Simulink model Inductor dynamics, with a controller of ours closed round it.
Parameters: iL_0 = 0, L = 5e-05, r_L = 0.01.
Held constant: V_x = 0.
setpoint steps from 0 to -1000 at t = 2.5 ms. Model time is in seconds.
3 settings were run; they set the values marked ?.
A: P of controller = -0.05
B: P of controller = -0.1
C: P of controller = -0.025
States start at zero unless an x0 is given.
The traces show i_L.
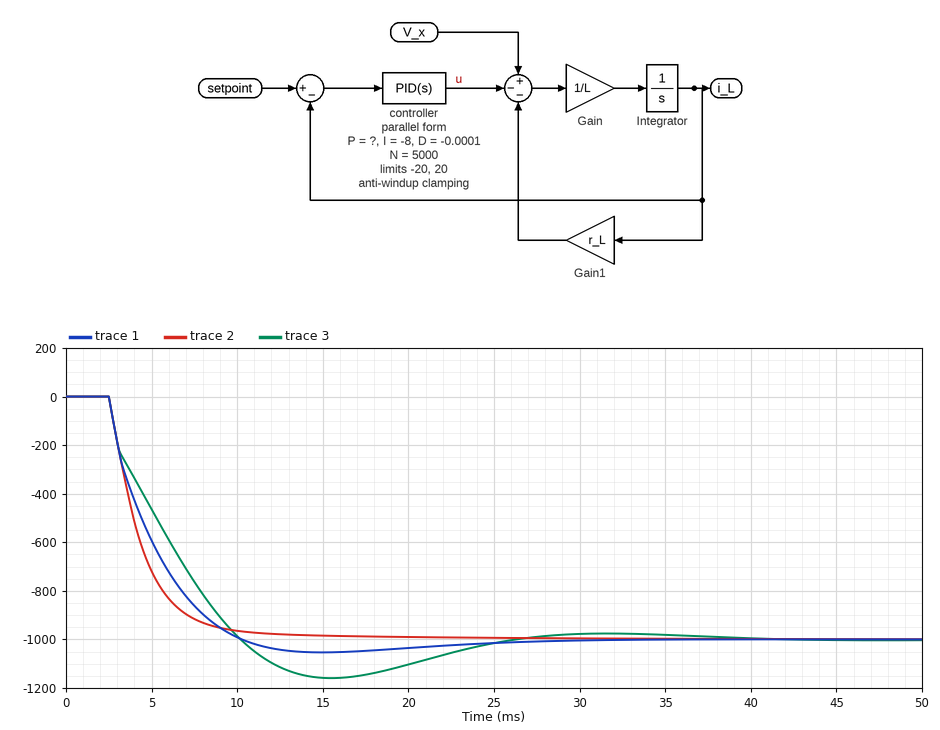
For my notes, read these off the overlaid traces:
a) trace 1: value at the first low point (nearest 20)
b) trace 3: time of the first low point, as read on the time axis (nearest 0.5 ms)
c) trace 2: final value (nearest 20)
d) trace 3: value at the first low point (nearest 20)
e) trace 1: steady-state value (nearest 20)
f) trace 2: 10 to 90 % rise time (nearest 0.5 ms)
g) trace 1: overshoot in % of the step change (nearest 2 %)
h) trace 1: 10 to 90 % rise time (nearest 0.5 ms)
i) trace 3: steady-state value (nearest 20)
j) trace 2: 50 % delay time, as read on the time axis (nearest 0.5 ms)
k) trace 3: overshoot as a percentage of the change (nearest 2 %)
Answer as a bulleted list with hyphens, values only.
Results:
- -1060
- 15.5 ms
- -1000
- -1160
- -1000
- 4.5 ms
- 6 %
- 5.5 ms
- -1000
- 4.0 ms
- 16 %
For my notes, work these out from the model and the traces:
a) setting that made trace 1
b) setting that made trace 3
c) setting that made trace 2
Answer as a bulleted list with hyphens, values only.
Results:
- A
- C
- B
